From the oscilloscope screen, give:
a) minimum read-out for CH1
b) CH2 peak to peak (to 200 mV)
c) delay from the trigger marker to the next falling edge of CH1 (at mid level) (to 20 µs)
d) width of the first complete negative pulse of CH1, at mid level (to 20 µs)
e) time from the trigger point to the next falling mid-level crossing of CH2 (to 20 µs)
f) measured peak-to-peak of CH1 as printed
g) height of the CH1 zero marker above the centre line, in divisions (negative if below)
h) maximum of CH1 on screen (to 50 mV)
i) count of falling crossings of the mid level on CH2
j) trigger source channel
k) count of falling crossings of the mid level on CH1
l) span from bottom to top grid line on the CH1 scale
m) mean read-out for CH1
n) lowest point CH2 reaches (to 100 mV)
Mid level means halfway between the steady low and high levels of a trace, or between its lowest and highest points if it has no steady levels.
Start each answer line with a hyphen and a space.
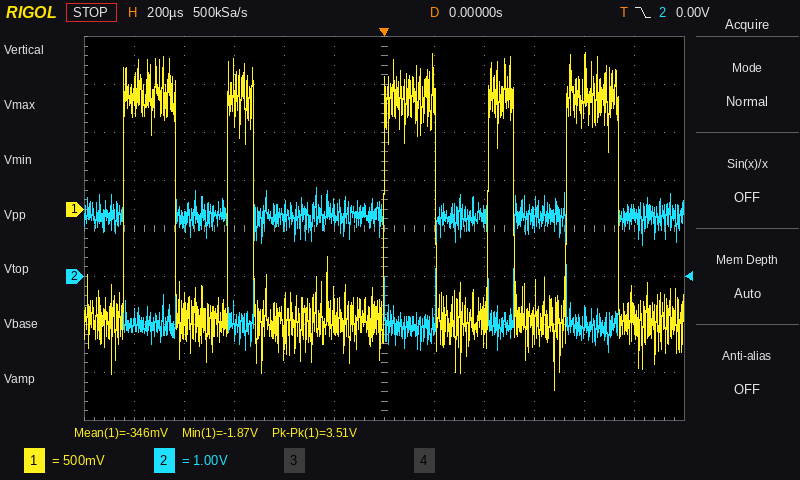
- -1.87 V
- 3.4 V
- 200 µs
- 200 µs
- 420 µs
- 3.51 V
- +0.4 div
- 1.65 V
- 5
- CH2
- 5
- 4 V
- -346 mV
- -1.6 V
